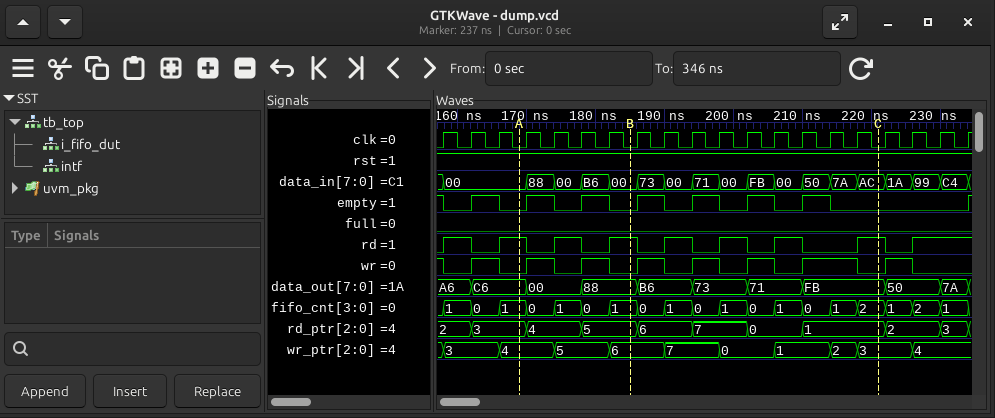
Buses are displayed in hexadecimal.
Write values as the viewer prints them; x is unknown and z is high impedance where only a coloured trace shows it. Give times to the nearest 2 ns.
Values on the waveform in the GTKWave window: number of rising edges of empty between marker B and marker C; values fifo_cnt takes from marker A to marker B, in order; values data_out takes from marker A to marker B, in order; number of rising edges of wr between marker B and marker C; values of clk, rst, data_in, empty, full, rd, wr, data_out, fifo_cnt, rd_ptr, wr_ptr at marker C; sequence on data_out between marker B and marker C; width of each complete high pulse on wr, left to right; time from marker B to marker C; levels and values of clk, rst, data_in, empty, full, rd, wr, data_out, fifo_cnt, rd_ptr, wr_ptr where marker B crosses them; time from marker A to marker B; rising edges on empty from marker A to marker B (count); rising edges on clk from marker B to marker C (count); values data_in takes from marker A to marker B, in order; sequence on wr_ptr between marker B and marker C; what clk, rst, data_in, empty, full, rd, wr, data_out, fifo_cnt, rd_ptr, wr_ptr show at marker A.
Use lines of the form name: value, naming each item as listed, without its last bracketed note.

number of rising edges of empty between marker B and marker C: 4
values fifo_cnt takes from marker A to marker B, in order: 1, 0, 1, 0, 1
values data_out takes from marker A to marker B, in order: C6, 00, 88
number of rising edges of wr between marker B and marker C: 4
values of clk, rst, data_in, empty, full, rd, wr, data_out, fifo_cnt, rd_ptr, wr_ptr at marker C: clk=0, rst=1, data_in=AC, empty=0, full=0, rd=1, wr=0, data_out=FB, fifo_cnt=2, rd_ptr=1, wr_ptr=3
sequence on data_out between marker B and marker C: 88, B6, 73, 71, FB
width of each complete high pulse on wr, left to right: 4 ns, 4 ns, 4 ns, 4 ns, 4 ns, 4 ns, 8 ns, 4 ns
time from marker B to marker C: 36 ns
levels and values of clk, rst, data_in, empty, full, rd, wr, data_out, fifo_cnt, rd_ptr, wr_ptr where marker B crosses them: clk=0, rst=1, data_in=00, empty=0, full=0, rd=1, wr=0, data_out=88, fifo_cnt=1, rd_ptr=5, wr_ptr=6
time from marker A to marker B: 16 ns
rising edges on empty from marker A to marker B: 2
rising edges on clk from marker B to marker C: 9
values data_in takes from marker A to marker B, in order: 00, 88, 00, B6, 00
sequence on wr_ptr between marker B and marker C: 6, 7, 0, 1, 2, 3
what clk, rst, data_in, empty, full, rd, wr, data_out, fifo_cnt, rd_ptr, wr_ptr show at marker A: clk=0, rst=1, data_in=00, empty=0, full=0, rd=1, wr=0, data_out=C6, fifo_cnt=1, rd_ptr=3, wr_ptr=4
